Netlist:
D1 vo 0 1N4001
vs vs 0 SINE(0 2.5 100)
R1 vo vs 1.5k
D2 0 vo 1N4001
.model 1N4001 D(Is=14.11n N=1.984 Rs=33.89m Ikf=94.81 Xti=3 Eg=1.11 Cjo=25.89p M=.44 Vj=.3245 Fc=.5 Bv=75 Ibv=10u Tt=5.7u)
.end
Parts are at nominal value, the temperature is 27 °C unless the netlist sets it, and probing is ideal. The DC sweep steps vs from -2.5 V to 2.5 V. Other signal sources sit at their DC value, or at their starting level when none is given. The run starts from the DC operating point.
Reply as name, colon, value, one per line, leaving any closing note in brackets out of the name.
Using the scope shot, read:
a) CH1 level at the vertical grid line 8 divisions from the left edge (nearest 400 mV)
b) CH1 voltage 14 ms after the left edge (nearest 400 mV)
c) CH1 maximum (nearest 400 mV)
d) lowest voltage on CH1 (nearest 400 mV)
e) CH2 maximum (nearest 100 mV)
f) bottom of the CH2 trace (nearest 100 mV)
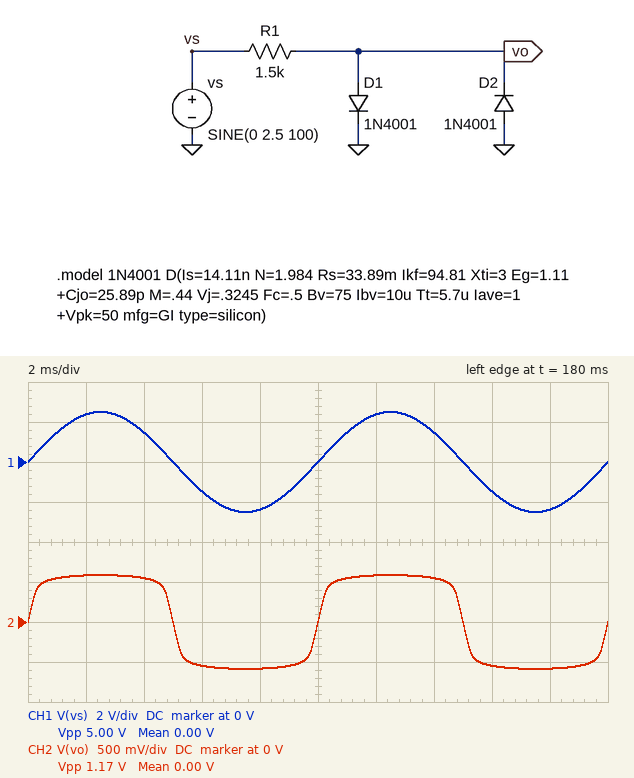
CH1 level at the vertical grid line 8 divisions from the left edge: -1.6 V
CH1 voltage 14 ms after the left edge: 1.6 V
CH1 maximum: 2.4 V
lowest voltage on CH1: -2.4 V
CH2 maximum: 600 mV
bottom of the CH2 trace: -600 mV
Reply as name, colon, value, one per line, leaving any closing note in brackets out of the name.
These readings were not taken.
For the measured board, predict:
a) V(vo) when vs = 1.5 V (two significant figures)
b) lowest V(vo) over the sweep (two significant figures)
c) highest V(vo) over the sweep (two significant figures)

V(vo) when vs = 1.5 V: 550 mV
lowest V(vo) over the sweep: -590 mV
highest V(vo) over the sweep: 590 mV
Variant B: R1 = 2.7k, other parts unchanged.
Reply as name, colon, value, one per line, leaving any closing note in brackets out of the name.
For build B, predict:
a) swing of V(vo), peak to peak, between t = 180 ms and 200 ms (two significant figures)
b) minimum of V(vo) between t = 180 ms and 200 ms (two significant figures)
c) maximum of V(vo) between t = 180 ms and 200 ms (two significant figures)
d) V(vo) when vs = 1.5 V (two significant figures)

swing of V(vo), peak to peak, between t = 180 ms and 200 ms: 1.1 V
minimum of V(vo) between t = 180 ms and 200 ms: -560 mV
maximum of V(vo) between t = 180 ms and 200 ms: 560 mV
V(vo) when vs = 1.5 V: 520 mV
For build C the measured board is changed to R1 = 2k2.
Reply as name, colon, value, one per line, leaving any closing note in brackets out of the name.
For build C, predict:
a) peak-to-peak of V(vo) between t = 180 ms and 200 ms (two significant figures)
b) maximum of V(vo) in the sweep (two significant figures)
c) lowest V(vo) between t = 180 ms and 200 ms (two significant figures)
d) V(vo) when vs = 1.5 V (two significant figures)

peak-to-peak of V(vo) between t = 180 ms and 200 ms: 1.1 V
maximum of V(vo) in the sweep: 570 mV
lowest V(vo) between t = 180 ms and 200 ms: -570 mV
V(vo) when vs = 1.5 V: 530 mV
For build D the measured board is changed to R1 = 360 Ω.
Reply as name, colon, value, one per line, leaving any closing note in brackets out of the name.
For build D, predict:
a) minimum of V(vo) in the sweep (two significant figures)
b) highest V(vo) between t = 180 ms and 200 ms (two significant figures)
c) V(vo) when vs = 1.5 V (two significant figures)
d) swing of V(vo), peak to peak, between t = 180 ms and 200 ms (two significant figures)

minimum of V(vo) in the sweep: -660 mV
highest V(vo) between t = 180 ms and 200 ms: 660 mV
V(vo) when vs = 1.5 V: 620 mV
swing of V(vo), peak to peak, between t = 180 ms and 200 ms: 1.3 V
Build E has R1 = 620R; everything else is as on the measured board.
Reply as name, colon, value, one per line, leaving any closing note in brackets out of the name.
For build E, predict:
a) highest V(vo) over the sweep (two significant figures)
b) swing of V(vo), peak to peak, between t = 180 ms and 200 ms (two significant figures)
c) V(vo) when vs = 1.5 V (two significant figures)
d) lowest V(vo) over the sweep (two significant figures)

highest V(vo) over the sweep: 630 mV
swing of V(vo), peak to peak, between t = 180 ms and 200 ms: 1.3 V
V(vo) when vs = 1.5 V: 590 mV
lowest V(vo) over the sweep: -630 mV
